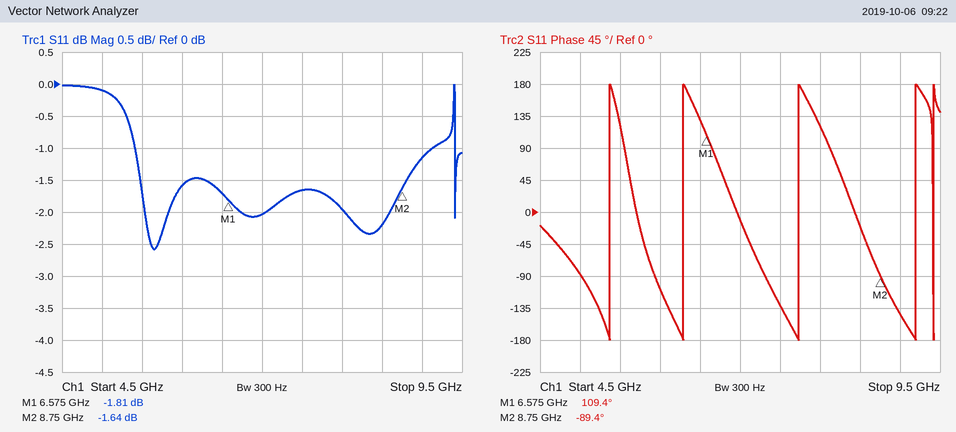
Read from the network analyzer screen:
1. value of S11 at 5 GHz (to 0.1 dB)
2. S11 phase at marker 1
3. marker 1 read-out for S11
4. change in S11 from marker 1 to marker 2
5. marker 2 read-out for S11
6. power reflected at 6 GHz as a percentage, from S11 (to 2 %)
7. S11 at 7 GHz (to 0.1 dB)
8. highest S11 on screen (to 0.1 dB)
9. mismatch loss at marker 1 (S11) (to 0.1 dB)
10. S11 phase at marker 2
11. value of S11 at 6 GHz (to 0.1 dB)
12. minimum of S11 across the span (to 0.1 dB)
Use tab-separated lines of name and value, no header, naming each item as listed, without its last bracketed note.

value of S11 at 5 GHz	-0.1 dB
S11 phase at marker 1	109.4°
marker 1 read-out for S11	-1.81 dB
change in S11 from marker 1 to marker 2	0.17 dB
marker 2 read-out for S11	-1.64 dB
power reflected at 6 GHz as a percentage, from S11	70 %
S11 at 7 GHz	-2.0 dB
highest S11 on screen	0.0 dB
mismatch loss at marker 1 (S11)	4.7 dB
S11 phase at marker 2	-89.4°
value of S11 at 6 GHz	-1.6 dB
minimum of S11 across the span	-2.6 dB
